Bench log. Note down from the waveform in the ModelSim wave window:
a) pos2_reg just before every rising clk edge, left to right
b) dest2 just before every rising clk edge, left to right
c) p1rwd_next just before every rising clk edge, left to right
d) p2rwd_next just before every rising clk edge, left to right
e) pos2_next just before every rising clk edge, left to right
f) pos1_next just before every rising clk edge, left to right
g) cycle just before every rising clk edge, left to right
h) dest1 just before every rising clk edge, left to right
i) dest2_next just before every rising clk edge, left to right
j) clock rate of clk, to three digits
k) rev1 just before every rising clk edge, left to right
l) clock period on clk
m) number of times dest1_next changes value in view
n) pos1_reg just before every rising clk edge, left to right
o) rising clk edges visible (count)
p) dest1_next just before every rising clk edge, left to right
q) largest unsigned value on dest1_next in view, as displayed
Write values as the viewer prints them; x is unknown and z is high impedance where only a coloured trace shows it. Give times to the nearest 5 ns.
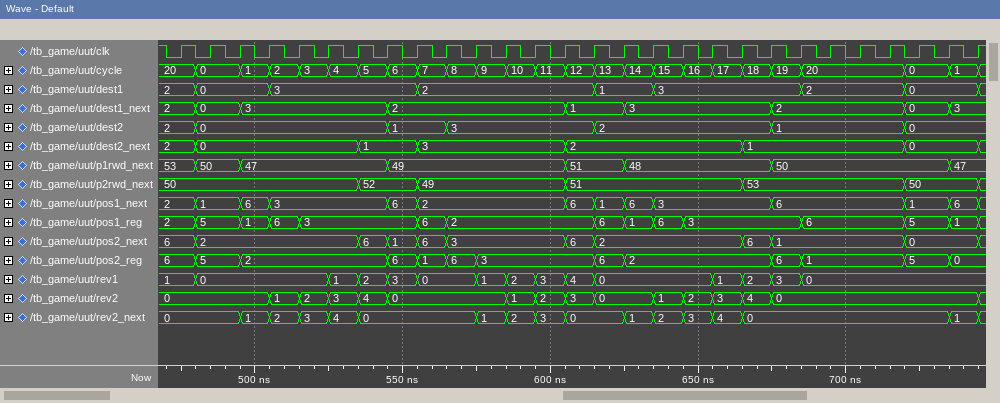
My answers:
6, 5, 5, 2, 2, 2, 2, 2, 6, 1, 6, 3, 3, 3, 3, 6, 2, 2, 2, 2, 2, 6, 1, 1, 1, 5, 5, 0
2, 0, 0, 0, 0, 0, 0, 0, 1, 1, 3, 3, 3, 3, 3, 2, 2, 2, 2, 2, 2, 1, 1, 1, 1, 0, 0, 0
53, 50, 50, 47, 47, 47, 47, 47, 49, 49, 49, 49, 49, 49, 51, 51, 48, 48, 48, 48, 48, 50, 50, 50, 50, 50, 50, 47
50, 50, 50, 50, 50, 50, 50, 52, 52, 49, 49, 49, 49, 49, 51, 51, 51, 51, 51, 51, 53, 53, 53, 53, 53, 50, 50, 50
6, 2, 2, 2, 2, 2, 2, 6, 1, 6, 3, 3, 3, 3, 6, 2, 2, 2, 2, 2, 6, 1, 1, 1, 1, 0, 0, 0
2, 1, 1, 6, 3, 3, 3, 3, 6, 2, 2, 2, 2, 2, 6, 1, 6, 3, 3, 3, 3, 6, 6, 6, 6, 1, 1, 6
20, 0, 0, 1, 2, 3, 4, 5, 6, 7, 8, 9, 10, 11, 12, 13, 14, 15, 16, 17, 18, 19, 20, 20, 20, 0, 0, 1
2, 0, 0, 0, 3, 3, 3, 3, 3, 2, 2, 2, 2, 2, 2, 1, 1, 3, 3, 3, 3, 3, 2, 2, 2, 0, 0, 0
2, 0, 0, 0, 0, 0, 0, 1, 1, 3, 3, 3, 3, 3, 2, 2, 2, 2, 2, 2, 1, 1, 1, 1, 1, 0, 0, 0
100 MHz
1, 0, 0, 0, 0, 0, 1, 2, 3, 0, 0, 1, 2, 3, 4, 0, 0, 0, 0, 1, 2, 3, 0, 0, 0, 0, 0, 0
10 ns
8
2, 5, 5, 1, 6, 3, 3, 3, 3, 6, 2, 2, 2, 2, 2, 6, 1, 6, 3, 3, 3, 3, 6, 6, 6, 5, 5, 1
28
2, 0, 0, 3, 3, 3, 3, 3, 2, 2, 2, 2, 2, 2, 1, 1, 3, 3, 3, 3, 3, 2, 2, 2, 2, 0, 0, 3
3
